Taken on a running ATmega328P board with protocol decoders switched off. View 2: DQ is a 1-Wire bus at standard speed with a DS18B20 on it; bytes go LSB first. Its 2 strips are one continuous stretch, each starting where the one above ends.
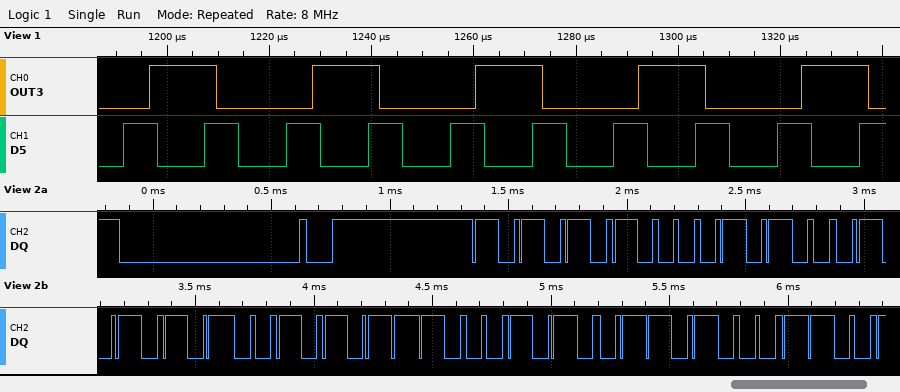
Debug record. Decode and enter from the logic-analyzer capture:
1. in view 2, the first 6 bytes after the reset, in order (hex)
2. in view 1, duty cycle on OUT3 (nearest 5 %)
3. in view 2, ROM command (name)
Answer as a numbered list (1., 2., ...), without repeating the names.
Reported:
1. 55 28 AA D4 51 16
2. 40 %
3. Match ROM
